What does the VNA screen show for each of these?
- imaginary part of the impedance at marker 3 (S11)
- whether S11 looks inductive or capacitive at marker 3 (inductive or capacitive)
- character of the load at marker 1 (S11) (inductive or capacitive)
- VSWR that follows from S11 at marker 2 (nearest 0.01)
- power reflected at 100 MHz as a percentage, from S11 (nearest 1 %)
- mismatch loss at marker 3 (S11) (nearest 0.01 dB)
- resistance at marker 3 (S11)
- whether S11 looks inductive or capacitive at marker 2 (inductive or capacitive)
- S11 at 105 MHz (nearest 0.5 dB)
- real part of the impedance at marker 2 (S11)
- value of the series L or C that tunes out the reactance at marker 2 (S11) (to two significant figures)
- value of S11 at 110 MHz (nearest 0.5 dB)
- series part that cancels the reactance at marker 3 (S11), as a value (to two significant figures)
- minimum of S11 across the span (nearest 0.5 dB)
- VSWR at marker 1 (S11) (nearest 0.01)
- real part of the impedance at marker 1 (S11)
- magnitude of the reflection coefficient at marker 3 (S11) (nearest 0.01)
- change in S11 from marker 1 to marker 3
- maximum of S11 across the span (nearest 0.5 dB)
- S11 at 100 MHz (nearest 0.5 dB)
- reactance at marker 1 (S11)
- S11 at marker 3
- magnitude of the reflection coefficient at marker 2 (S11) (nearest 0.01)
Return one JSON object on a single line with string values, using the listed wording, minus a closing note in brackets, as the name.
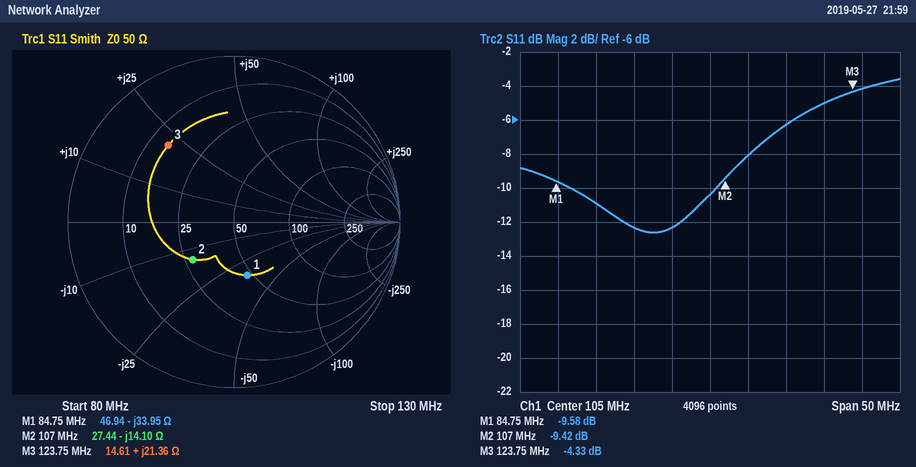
{"imaginary part of the impedance at marker 3": "+21.36 Ω", "whether S11 looks inductive or capacitive at marker 3": "inductive", "character of the load at marker 1 (S11)": "capacitive", "VSWR that follows from S11 at marker 2": "2.02", "power reflected at 100 MHz as a percentage, from S11": "6 %", "mismatch loss at marker 3 (S11)": "2.00 dB", "resistance at marker 3": "14.61 Ω", "whether S11 looks inductive or capacitive at marker 2": "capacitive", "S11 at 105 MHz": "-10.5 dB", "real part of the impedance at marker 2": "27.44 Ω", "value of the series L or C that tunes out the reactance at marker 2 (S11)": "21 nH", "value of S11 at 110 MHz": "-8.0 dB", "series part that cancels the reactance at marker 3 (S11), as a value": "60 pF", "minimum of S11 across the span": "-12.5 dB", "VSWR at marker 1 (S11)": "1.99", "real part of the impedance at marker 1": "46.94 Ω", "magnitude of the reflection coefficient at marker 3 (S11)": "0.61", "change in S11 from marker 1 to marker 3": "5.25 dB", "maximum of S11 across the span": "-3.5 dB", "S11 at 100 MHz": "-12.5 dB", "reactance at marker 1": "-33.95 Ω", "S11 at marker 3": "-4.33 dB", "magnitude of the reflection coefficient at marker 2 (S11)": "0.34"}
